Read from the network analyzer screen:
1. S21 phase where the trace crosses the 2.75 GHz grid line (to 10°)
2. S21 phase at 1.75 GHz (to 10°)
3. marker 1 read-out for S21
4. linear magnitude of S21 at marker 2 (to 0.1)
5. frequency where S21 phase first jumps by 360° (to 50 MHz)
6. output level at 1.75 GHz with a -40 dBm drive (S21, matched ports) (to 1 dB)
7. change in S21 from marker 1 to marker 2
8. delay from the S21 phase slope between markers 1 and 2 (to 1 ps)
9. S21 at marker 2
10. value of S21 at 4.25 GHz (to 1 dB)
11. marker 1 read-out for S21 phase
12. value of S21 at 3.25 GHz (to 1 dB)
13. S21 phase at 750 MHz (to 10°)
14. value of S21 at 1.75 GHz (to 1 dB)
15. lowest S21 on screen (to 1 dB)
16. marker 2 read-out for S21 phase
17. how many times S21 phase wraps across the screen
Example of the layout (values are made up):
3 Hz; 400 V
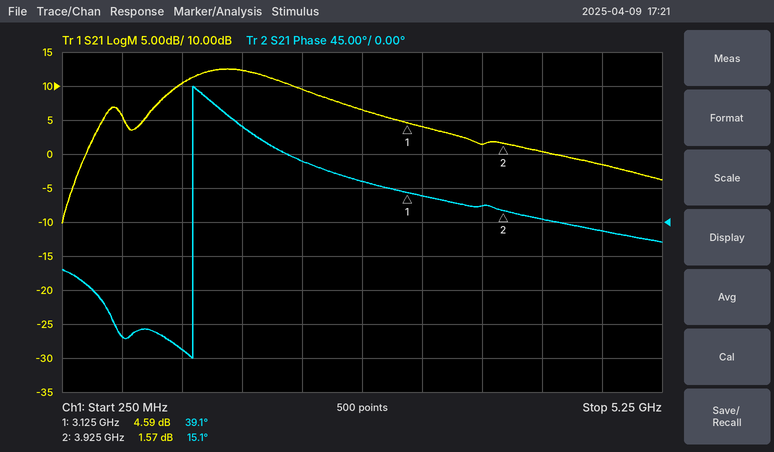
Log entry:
50°; 130°; 4.59 dB; 1.2; 1.35 GHz; -28 dBm; -3.02 dB; 83 ps; 1.57 dB; 0 dB; 39.1°; 4 dB; -150°; 12 dB; -10 dB; 15.1°; 1
